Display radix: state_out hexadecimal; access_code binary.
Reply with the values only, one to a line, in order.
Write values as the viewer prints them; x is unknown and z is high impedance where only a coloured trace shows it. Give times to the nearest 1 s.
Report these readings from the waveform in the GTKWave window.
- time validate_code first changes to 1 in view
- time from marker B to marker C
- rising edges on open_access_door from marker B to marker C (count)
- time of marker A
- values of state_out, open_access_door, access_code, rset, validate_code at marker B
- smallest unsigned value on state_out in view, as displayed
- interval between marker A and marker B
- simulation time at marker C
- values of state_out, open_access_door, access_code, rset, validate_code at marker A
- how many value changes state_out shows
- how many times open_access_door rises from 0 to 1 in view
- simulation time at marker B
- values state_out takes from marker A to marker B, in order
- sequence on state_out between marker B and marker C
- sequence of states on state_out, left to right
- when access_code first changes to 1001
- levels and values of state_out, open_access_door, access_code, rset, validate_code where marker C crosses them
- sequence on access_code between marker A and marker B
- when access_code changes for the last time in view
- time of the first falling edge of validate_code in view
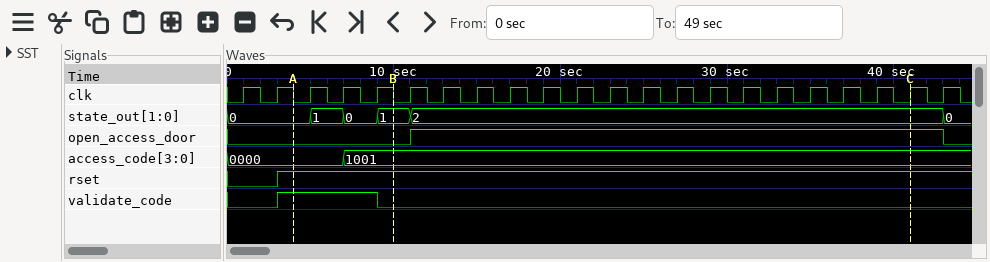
3 s
31 s
1
4 s
state_out=1, open_access_door=0, access_code=1001, rset=1, validate_code=0
0
6 s
41 s
state_out=0, open_access_door=0, access_code=0000, rset=1, validate_code=1
5
1
10 s
0, 1, 0, 1
1, 2
0, 1, 0, 1, 2, 0
7 s
state_out=2, open_access_door=1, access_code=1001, rset=1, validate_code=0
0000, 1001
7 s
9 s
